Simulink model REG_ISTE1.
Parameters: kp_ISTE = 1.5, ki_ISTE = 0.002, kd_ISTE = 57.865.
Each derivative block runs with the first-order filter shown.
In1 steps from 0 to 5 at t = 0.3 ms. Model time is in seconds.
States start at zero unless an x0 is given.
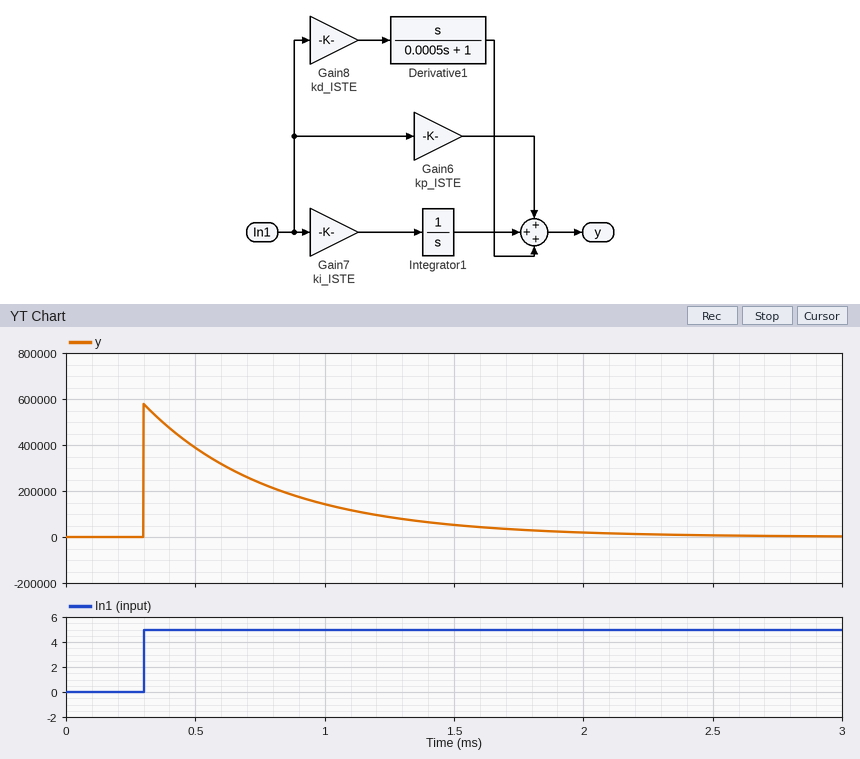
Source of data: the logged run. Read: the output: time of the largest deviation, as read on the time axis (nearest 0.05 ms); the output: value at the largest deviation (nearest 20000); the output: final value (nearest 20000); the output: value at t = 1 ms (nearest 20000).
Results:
0.30 ms
580000
0
140000
